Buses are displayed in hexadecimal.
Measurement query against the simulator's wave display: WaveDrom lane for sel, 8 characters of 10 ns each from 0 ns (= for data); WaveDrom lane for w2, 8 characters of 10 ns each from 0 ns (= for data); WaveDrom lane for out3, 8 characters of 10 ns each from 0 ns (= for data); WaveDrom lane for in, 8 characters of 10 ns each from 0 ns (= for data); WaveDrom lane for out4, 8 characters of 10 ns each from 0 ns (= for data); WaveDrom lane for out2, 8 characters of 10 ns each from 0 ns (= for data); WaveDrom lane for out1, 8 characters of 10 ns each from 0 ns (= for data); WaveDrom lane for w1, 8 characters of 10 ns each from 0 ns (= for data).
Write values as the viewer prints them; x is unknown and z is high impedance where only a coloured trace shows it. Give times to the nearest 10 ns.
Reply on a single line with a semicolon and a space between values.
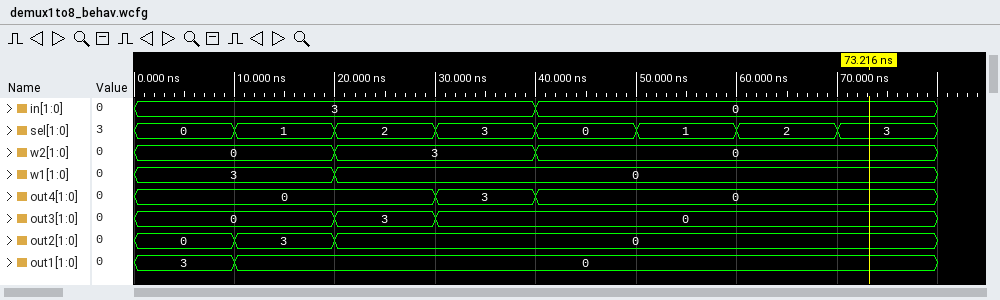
{name: 'sel', wave: '========', data: '0 1 2 3 0 1 2 3'}; {name: 'w2', wave: '=.=.=...', data: '0 3 0'}; {name: 'out3', wave: '=.==....', data: '0 3 0'}; {name: 'in', wave: '=...=...', data: '3 0'}; {name: 'out4', wave: '=..==...', data: '0 3 0'}; {name: 'out2', wave: '===.....', data: '0 3 0'}; {name: 'out1', wave: '==......', data: '3 0'}; {name: 'w1', wave: '=.=.....', data: '3 0'}
